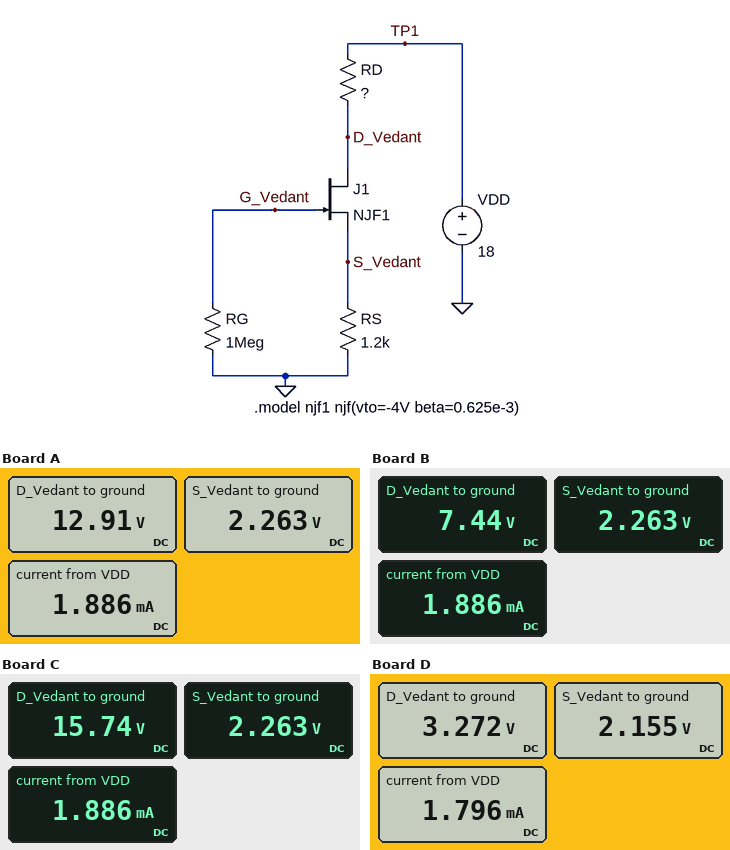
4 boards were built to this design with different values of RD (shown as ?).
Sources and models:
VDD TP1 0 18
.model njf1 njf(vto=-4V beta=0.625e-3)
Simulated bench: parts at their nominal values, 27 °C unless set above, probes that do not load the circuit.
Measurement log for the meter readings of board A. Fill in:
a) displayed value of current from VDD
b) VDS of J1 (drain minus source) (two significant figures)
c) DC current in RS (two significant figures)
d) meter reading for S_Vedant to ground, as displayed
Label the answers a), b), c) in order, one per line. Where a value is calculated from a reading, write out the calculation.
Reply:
a) 1.886 mA
b) 12.91 V - 2.263 V = 11 V
c) (2.263 V) / 1.2 kΩ = 1.9 mA
d) 2.263 V
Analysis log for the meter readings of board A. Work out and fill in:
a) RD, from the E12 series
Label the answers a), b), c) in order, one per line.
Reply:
a) 2.7 kΩ
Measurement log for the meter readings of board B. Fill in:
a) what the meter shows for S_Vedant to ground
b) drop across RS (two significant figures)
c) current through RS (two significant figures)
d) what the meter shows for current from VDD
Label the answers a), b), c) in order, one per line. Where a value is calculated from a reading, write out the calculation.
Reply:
a) 2.263 V
b) 2.263 V = 2.3 V
c) (2.263 V) / 1.2 kΩ = 1.9 mA
d) 1.886 mA
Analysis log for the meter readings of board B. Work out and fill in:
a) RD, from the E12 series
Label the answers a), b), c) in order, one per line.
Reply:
a) 5.6 kΩ
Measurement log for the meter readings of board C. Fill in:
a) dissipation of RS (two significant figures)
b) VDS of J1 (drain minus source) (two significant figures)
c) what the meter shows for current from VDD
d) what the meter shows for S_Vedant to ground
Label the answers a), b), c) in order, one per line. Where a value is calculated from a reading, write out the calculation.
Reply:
a) (2.263 V)^2 / 1.2 kΩ = 4.3 mW
b) 15.74 V - 2.263 V = 13 V
c) 1.886 mA
d) 2.263 V
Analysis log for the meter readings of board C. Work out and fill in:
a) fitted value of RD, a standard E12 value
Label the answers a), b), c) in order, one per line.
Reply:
a) 1.2 kΩ
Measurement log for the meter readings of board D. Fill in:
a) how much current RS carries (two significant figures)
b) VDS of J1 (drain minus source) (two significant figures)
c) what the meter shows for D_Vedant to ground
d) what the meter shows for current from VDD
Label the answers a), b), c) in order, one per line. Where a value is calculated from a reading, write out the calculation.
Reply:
a) (2.155 V) / 1.2 kΩ = 1.8 mA
b) 3.272 V - 2.155 V = 1.1 V
c) 3.272 V
d) 1.796 mA
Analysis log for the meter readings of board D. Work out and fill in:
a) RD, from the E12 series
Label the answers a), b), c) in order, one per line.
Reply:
a) 8.2 kΩ
